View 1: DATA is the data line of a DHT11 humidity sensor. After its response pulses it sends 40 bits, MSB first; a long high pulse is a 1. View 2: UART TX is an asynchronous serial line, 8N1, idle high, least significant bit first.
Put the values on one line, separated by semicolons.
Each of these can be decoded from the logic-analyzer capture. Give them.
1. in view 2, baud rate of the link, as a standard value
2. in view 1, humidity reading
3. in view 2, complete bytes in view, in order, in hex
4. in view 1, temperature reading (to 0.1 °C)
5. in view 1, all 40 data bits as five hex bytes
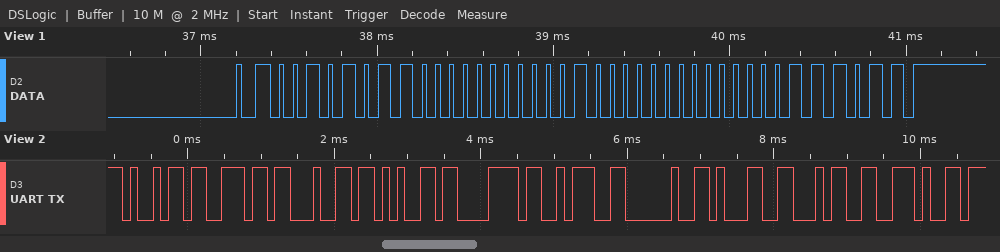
9600 baud; 43 %; 0x69 0x6E 0x64 0x65 0x78 0x3A 0x20 0x31 0x34 0x2E; 16.0 °C; 2B 00 10 00 3B
